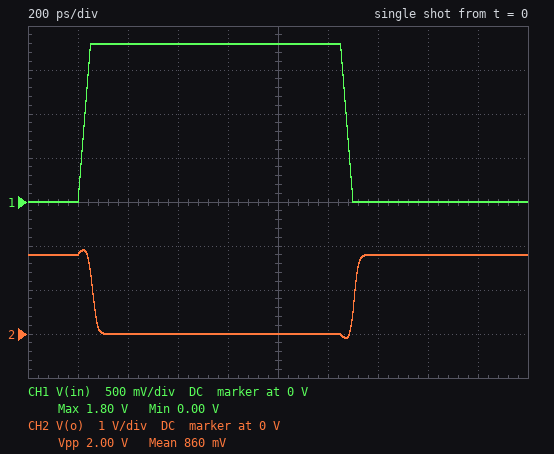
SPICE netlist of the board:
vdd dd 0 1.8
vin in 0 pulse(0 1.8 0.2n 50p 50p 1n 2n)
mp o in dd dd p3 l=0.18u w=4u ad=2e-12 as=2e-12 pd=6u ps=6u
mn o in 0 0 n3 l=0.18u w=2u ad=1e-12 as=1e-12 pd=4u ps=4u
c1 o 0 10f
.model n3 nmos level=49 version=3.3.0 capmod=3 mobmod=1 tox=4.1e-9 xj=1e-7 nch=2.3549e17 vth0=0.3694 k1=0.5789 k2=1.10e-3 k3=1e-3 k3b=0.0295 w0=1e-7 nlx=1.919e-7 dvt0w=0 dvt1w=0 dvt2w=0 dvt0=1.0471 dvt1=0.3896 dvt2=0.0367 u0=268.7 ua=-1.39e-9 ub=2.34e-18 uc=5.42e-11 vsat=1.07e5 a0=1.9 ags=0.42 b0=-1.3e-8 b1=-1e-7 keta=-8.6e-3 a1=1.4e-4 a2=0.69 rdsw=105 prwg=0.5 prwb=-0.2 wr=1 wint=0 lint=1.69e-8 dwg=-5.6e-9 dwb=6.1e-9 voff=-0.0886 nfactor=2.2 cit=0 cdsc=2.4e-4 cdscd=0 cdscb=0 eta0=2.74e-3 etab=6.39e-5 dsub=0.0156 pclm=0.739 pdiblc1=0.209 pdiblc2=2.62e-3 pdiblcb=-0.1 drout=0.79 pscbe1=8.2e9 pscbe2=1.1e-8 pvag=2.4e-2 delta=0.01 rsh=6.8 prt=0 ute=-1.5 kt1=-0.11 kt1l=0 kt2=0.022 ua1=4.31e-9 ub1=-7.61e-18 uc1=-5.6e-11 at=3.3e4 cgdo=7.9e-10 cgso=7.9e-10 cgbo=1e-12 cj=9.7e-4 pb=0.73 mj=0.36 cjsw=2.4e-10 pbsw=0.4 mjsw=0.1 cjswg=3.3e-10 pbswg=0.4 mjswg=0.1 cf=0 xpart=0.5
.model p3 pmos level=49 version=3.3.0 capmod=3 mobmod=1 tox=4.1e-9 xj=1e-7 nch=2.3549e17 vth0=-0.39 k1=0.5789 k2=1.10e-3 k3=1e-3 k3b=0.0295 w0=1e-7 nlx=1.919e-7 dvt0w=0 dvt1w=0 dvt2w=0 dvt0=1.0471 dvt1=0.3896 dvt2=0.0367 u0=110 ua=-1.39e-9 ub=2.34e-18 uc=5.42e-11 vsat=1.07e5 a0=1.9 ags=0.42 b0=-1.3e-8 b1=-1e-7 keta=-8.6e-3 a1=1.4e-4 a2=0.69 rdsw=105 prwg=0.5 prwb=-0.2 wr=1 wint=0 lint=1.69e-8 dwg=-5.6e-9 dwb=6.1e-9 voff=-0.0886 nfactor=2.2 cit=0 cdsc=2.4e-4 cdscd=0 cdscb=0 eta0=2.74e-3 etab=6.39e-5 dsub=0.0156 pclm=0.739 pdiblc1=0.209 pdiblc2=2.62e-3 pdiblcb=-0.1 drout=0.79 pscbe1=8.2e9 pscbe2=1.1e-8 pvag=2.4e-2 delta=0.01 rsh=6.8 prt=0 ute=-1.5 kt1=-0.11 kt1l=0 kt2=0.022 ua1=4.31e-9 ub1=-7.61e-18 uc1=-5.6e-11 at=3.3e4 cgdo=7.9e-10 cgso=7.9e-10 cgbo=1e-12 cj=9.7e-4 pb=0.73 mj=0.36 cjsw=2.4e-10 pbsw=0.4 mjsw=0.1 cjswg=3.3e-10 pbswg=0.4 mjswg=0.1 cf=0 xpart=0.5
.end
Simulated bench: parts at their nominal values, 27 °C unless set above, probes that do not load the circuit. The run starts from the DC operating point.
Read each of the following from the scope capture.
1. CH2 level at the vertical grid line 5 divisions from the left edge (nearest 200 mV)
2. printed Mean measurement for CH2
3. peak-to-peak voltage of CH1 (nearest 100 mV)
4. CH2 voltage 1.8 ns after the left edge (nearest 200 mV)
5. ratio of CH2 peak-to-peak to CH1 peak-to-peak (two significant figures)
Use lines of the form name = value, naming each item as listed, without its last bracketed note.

CH2 level at the vertical grid line 5 divisions from the left edge = 0 V
printed Mean measurement for CH2 = 860 mV
peak-to-peak voltage of CH1 = 1.8 V
CH2 voltage 1.8 ns after the left edge = 1.8 V
ratio of CH2 peak-to-peak to CH1 peak-to-peak = 1.1
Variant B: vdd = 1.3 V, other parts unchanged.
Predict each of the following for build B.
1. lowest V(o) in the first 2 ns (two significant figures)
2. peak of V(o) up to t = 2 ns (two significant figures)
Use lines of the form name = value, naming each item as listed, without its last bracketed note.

lowest V(o) in the first 2 ns = -180 mV
peak of V(o) up to t = 2 ns = 1.5 V
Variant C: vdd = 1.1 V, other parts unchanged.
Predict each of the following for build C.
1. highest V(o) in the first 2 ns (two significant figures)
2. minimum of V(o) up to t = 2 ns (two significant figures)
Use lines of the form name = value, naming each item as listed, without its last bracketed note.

highest V(o) in the first 2 ns = 1.3 V
minimum of V(o) up to t = 2 ns = -230 mV
